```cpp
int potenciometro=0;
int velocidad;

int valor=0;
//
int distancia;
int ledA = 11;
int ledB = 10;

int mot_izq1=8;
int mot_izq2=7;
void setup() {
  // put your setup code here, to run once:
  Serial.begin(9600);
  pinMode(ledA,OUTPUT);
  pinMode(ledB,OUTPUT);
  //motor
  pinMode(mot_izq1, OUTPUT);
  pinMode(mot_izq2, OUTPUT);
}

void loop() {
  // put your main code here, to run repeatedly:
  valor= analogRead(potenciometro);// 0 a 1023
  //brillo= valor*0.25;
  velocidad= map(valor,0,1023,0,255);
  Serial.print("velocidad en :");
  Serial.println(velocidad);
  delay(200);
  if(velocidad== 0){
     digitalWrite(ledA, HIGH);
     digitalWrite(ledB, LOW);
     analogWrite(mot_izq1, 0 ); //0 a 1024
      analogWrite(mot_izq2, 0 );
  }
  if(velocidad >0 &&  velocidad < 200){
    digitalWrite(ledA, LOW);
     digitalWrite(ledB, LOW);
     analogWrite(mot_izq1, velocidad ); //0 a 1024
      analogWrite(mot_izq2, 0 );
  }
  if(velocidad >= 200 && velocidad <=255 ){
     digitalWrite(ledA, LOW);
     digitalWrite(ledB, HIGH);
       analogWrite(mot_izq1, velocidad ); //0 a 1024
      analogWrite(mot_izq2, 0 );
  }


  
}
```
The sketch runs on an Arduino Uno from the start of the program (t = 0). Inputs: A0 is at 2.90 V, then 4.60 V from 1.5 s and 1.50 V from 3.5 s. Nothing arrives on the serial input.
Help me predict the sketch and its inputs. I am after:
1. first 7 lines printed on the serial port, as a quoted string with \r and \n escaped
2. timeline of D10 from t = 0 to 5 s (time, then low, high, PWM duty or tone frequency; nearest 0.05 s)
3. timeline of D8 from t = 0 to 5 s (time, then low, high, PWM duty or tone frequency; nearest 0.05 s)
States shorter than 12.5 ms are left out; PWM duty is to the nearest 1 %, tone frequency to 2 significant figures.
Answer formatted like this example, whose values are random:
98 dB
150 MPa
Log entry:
"velocidad en :147\r\nvelocidad en :147\r\nvelocidad en :147\r\nvelocidad en :147\r\nvelocidad en :147\r\nvelocidad en :147\r\nvelocidad en :147\r\n"
0 s low; 1.8 s high; 3.8 s low
0 s low; 0.2 s high; 3.8 s low
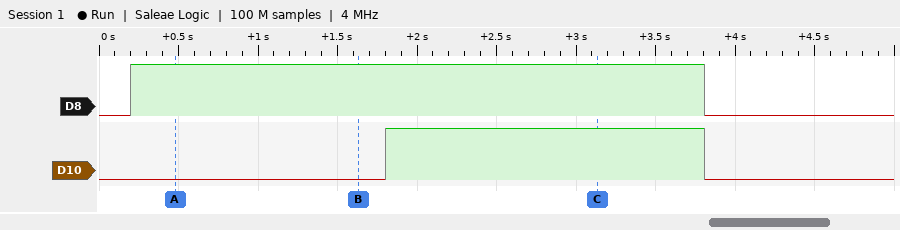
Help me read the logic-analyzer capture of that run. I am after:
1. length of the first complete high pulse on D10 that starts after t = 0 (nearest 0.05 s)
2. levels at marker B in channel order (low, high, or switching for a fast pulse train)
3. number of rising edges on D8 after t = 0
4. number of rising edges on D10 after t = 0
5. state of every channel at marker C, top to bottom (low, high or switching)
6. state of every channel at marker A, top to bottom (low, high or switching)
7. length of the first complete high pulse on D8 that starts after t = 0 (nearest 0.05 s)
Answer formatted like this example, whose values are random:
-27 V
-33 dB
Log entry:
2.00 s
D8 high, D10 low
1
1
D8 high, D10 high
D8 high, D10 low
3.60 s
